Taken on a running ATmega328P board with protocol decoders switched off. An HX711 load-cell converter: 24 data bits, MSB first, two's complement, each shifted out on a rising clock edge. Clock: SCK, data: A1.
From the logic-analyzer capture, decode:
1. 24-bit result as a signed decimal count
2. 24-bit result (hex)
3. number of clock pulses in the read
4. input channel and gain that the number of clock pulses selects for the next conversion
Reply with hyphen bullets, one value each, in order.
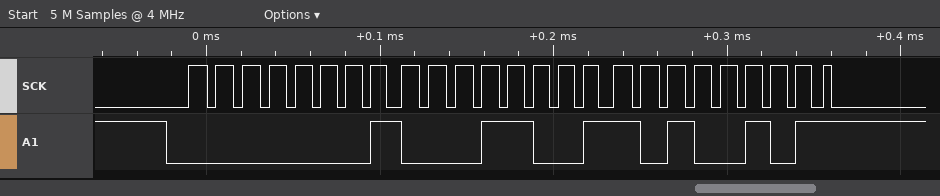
- 72101
- 0x0119A5
- 25
- channel A, gain 128
